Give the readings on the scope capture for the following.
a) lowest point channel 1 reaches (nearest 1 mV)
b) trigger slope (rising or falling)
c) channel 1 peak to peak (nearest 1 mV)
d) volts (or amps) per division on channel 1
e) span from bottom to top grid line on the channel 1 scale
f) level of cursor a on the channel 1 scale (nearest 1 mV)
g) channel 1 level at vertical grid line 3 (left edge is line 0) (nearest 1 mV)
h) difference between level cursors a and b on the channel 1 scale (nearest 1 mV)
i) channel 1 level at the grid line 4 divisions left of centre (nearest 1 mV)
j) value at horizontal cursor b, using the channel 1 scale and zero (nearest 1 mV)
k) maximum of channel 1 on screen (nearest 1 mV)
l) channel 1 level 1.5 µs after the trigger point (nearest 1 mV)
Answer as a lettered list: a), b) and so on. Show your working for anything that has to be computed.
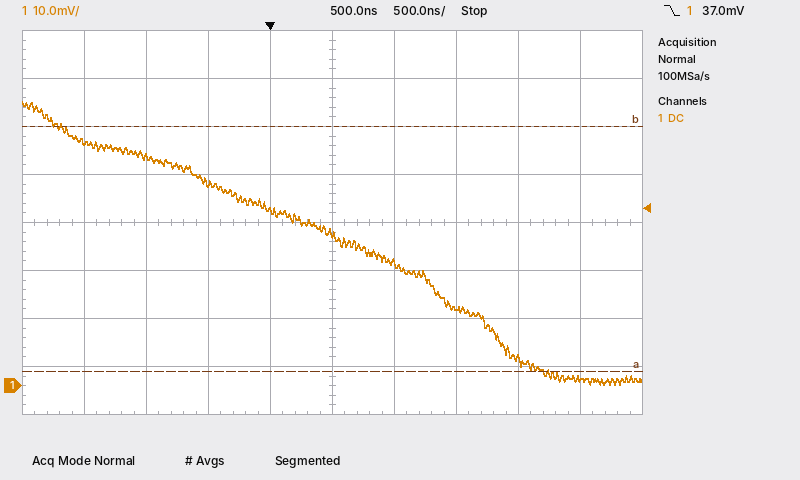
a) 0 mV
b) falling
c) 59 mV − (0 mV) = 59 mV
d) 10 mV
e) 80 mV
f) 3 mV
g) 42 mV
h) 51 mV
i) 51 mV
j) 54 mV
k) 59 mV
l) 16 mV
